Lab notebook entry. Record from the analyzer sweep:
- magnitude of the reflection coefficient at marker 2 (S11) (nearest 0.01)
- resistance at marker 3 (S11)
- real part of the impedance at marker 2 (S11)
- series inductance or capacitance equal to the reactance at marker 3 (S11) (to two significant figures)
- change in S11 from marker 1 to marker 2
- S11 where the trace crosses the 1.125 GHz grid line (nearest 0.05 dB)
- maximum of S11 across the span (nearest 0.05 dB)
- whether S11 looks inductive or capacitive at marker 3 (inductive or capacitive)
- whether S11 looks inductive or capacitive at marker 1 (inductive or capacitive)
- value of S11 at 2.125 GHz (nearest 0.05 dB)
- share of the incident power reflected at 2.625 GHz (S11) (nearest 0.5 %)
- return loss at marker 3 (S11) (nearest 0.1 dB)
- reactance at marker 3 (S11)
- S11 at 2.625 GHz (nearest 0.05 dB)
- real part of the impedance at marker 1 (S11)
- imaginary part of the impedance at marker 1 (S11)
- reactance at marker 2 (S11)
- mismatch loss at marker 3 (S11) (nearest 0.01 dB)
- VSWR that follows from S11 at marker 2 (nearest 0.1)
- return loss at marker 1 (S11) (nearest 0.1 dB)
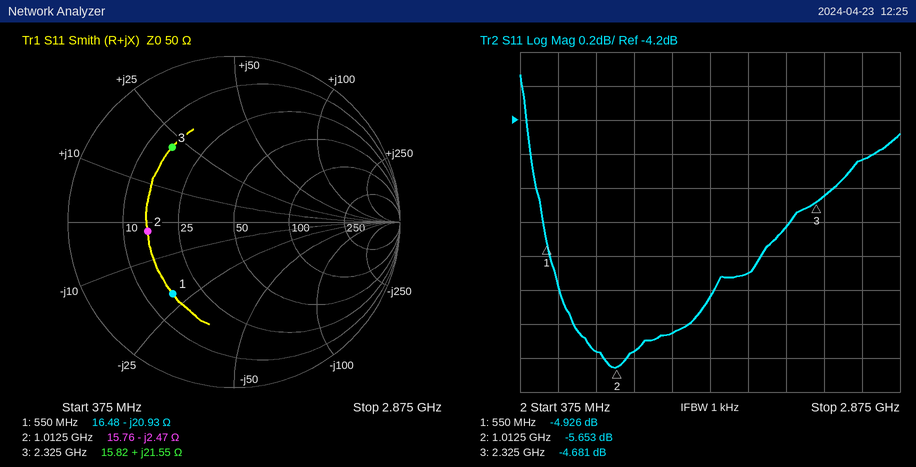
0.52
15.82 Ω
15.76 Ω
1.5 nH
-0.727 dB
-5.55 dB
-3.95 dB
inductive
capacitive
-4.85 dB
36.0 %
4.7 dB
+21.55 Ω
-4.45 dB
16.48 Ω
-20.93 Ω
-2.47 Ω
1.81 dB
3.2
4.9 dB
